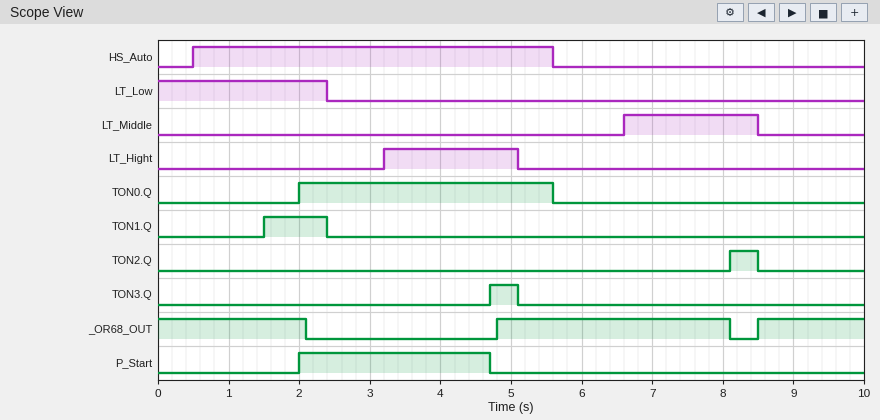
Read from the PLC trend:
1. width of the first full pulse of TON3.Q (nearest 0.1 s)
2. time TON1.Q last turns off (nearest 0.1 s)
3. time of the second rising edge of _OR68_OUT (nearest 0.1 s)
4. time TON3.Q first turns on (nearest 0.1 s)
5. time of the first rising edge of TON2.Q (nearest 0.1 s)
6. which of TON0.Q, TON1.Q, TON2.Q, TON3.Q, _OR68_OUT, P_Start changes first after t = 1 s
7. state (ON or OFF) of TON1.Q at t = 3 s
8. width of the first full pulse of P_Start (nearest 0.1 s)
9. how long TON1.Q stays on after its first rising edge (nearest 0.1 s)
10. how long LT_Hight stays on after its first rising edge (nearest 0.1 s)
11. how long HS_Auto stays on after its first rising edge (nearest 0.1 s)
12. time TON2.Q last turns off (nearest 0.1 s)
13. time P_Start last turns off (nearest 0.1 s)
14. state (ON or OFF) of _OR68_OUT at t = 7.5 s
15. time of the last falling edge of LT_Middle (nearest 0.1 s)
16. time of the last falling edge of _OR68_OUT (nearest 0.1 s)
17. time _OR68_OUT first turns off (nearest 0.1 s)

0.4 s
2.4 s
8.5 s
4.7 s
8.1 s
TON1.Q
OFF
2.7 s
0.9 s
1.9 s
5.1 s
8.5 s
4.7 s
ON
8.5 s
8.1 s
2.1 s
